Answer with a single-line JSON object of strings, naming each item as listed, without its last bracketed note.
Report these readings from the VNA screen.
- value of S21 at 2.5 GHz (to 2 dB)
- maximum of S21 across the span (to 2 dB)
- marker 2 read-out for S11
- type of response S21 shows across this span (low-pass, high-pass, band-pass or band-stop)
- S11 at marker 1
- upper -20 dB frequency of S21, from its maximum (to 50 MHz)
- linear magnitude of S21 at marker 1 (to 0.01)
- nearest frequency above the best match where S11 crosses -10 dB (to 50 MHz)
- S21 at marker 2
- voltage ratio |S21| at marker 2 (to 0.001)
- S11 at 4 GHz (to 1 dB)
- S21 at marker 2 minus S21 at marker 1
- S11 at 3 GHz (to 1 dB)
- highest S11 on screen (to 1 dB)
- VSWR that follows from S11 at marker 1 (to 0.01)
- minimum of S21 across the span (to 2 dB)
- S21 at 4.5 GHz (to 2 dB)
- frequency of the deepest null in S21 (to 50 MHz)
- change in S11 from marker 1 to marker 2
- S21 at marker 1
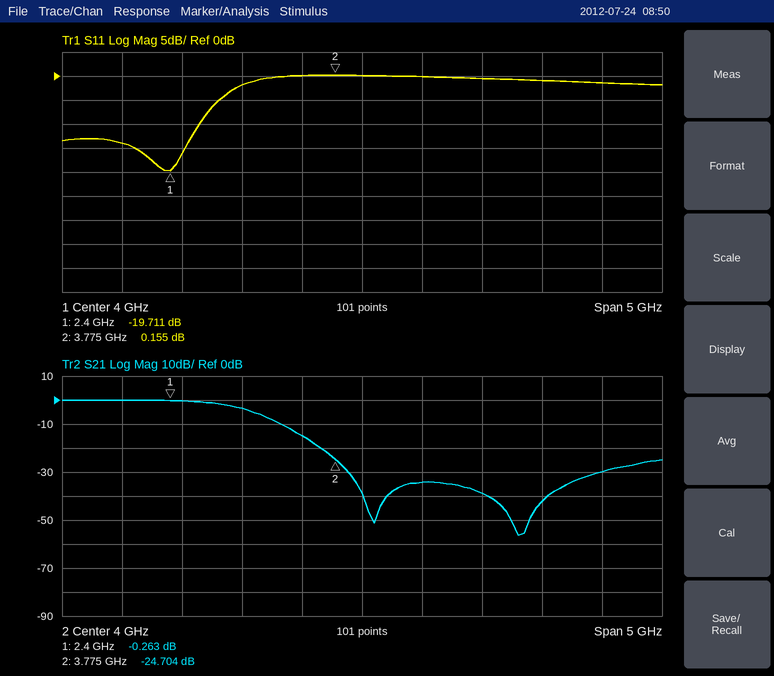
{"value of S21 at 2.5 GHz": "0 dB", "maximum of S21 across the span": "0 dB", "marker 2 read-out for S11": "0.155 dB", "type of response S21 shows across this span": "low-pass", "S11 at marker 1": "-19.711 dB", "upper -20 dB frequency of S21, from its maximum": "3.65 GHz", "linear magnitude of S21 at marker 1": "0.97", "nearest frequency above the best match where S11 crosses -10 dB": "2.65 GHz", "S21 at marker 2": "-24.704 dB", "voltage ratio |S21| at marker 2": "0.058", "S11 at 4 GHz": "0 dB", "S21 at marker 2 minus S21 at marker 1": "-24.441 dB", "S11 at 3 GHz": "-2 dB", "highest S11 on screen": "0 dB", "VSWR that follows from S11 at marker 1": "1.23", "minimum of S21 across the span": "-56 dB", "S21 at 4.5 GHz": "-34 dB", "frequency of the deepest null in S21": "5.30 GHz", "change in S11 from marker 1 to marker 2": "19.866 dB", "S21 at marker 1": "-0.263 dB"}
